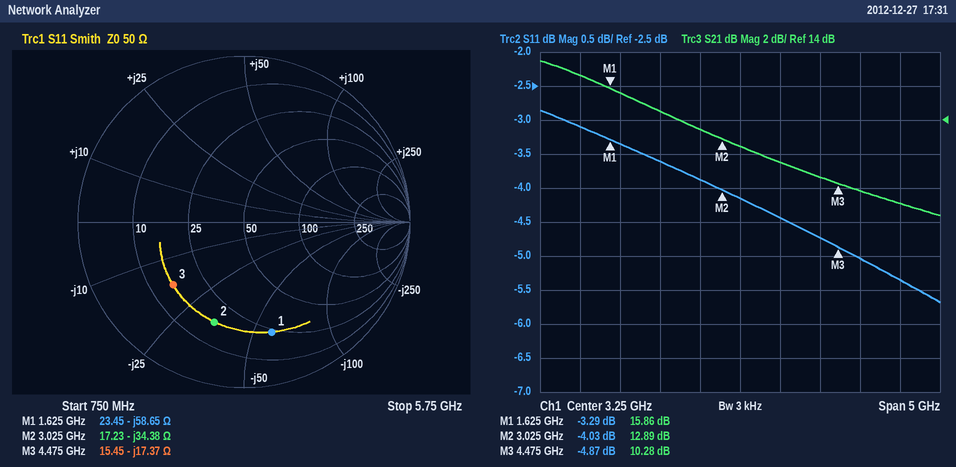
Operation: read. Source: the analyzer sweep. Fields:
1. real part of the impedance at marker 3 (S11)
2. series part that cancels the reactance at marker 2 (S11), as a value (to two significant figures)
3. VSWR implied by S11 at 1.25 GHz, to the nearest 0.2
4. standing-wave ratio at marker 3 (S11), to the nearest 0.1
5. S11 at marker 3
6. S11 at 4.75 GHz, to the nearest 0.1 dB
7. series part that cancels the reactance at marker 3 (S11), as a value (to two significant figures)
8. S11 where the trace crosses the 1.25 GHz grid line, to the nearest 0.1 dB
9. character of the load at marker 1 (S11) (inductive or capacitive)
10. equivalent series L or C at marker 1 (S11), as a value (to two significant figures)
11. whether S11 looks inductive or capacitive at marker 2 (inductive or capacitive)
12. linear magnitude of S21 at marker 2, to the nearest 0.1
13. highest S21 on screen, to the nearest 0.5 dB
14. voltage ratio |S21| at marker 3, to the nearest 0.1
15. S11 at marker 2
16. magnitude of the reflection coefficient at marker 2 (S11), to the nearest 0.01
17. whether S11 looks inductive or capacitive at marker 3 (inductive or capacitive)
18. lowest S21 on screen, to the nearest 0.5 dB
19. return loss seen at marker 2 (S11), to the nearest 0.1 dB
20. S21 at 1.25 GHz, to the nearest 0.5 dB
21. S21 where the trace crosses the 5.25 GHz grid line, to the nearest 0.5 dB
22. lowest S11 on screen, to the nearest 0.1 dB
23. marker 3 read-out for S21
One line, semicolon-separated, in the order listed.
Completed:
15.45 Ω; 1.8 nH; 5.6; 3.7; -4.87 dB; -5.0 dB; 620 pH; -3.1 dB; capacitive; 1.7 pF; capacitive; 4.4; 17.5 dB; 3.3; -4.03 dB; 0.63; capacitive; 8.5 dB; 4.0 dB; 16.5 dB; 9.0 dB; -5.7 dB; 10.28 dB
